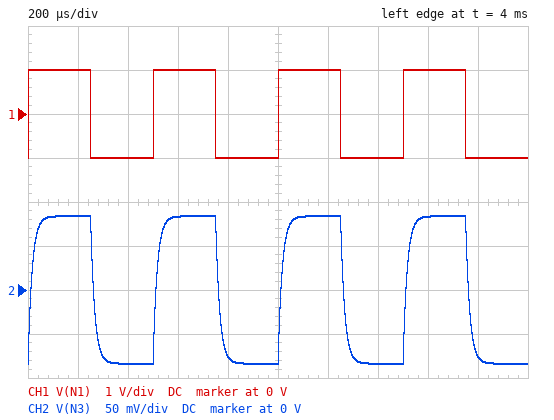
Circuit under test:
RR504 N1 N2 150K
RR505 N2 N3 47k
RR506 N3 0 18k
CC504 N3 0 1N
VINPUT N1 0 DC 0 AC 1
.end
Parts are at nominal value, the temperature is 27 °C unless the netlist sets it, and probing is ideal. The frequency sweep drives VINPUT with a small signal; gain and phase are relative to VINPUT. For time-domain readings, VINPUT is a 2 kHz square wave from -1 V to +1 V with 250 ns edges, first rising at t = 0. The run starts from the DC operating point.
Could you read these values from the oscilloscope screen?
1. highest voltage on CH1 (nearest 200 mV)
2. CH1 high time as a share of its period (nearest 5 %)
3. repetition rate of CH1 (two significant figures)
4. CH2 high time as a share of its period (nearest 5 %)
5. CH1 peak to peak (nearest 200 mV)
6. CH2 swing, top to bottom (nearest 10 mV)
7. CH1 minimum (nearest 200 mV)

1.0 V
50 %
2.0 kHz
50 %
2.0 V
170 mV
-1.0 V
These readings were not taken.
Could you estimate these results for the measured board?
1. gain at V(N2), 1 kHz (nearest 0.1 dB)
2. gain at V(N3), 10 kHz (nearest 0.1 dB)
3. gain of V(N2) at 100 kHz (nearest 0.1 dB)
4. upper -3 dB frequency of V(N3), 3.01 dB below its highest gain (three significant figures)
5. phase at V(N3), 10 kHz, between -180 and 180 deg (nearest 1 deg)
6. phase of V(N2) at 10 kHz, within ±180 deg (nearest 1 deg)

-10.4 dB
-24.7 dB
-12.4 dB
9.65 kHz
-46 deg
-7 deg
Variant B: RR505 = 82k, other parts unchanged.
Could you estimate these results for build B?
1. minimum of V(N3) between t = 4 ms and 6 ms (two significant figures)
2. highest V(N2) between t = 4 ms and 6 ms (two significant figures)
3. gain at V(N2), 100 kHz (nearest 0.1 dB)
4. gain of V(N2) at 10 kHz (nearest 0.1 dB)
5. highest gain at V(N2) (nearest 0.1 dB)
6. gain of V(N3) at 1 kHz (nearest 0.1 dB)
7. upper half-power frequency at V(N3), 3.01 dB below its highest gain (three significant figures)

-72 mV
400 mV
-9.0 dB
-8.5 dB
-8.0 dB
-22.9 dB
9.53 kHz
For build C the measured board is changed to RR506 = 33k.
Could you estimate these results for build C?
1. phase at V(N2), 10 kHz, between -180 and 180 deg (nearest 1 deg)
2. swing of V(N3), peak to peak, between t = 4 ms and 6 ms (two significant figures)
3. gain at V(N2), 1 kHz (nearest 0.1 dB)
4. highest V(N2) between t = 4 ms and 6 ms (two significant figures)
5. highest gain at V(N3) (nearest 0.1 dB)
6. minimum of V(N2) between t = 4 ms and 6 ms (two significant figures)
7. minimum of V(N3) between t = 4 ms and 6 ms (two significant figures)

-10 deg
290 mV
-9.2 dB
350 mV
-16.9 dB
-350 mV
-140 mV
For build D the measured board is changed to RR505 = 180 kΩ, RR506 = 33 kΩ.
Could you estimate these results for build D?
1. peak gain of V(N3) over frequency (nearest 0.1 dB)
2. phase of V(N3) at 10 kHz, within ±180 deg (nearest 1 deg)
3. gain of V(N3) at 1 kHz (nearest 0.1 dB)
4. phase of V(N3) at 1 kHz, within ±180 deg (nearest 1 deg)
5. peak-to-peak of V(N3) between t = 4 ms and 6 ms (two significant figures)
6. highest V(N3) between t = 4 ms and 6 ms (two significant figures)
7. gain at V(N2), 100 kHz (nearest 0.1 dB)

-20.8 dB
-62 deg
-21.0 dB
-11 deg
180 mV
91 mV
-5.3 dB
